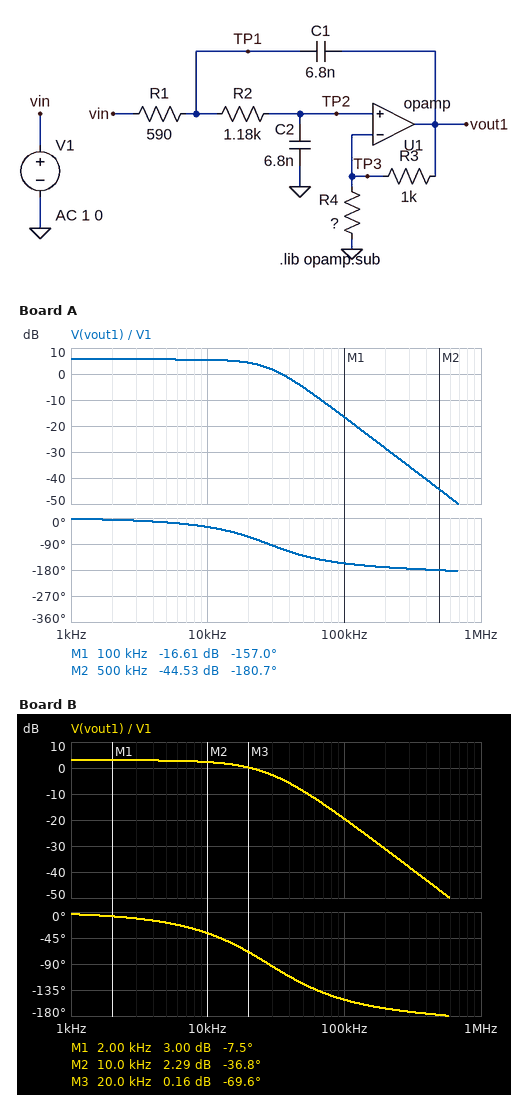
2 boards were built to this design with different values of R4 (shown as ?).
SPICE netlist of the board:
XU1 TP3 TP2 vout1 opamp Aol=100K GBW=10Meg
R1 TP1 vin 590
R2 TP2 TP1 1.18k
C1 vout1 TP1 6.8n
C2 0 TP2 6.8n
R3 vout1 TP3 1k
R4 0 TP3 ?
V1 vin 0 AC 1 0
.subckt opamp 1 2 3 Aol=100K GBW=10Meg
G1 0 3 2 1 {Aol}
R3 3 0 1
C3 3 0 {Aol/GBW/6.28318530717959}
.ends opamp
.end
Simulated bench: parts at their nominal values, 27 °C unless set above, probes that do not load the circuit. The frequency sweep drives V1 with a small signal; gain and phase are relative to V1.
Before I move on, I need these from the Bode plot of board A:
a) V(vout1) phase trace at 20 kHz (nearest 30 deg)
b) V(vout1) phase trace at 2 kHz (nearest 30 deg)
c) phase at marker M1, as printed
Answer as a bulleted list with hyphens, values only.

- -60 deg
- 0 deg
- -157.0 deg
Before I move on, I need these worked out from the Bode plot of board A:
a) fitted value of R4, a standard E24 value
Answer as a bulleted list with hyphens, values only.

- 1.1 kΩ
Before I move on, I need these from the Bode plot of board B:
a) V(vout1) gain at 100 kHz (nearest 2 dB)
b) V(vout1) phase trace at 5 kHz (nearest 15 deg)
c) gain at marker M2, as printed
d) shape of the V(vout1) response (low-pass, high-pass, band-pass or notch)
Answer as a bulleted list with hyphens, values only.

- -20 dB
- -15 deg
- 2.29 dB
- low-pass
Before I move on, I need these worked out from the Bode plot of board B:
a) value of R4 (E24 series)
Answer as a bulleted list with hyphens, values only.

- 2.4 kΩ
